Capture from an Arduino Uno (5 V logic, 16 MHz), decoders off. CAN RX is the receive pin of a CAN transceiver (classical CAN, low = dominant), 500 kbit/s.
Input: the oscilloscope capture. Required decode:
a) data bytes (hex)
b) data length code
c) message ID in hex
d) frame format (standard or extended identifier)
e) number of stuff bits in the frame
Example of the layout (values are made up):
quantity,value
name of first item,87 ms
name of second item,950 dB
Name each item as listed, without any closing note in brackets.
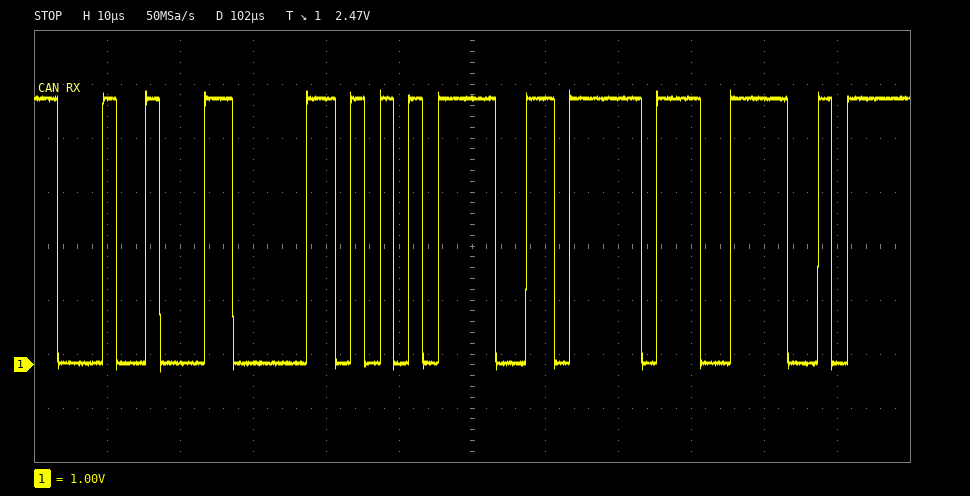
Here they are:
quantity,value
data bytes,AB CD
data length code,2
message ID in hex,0x123
frame format,standard
number of stuff bits in the frame,2
